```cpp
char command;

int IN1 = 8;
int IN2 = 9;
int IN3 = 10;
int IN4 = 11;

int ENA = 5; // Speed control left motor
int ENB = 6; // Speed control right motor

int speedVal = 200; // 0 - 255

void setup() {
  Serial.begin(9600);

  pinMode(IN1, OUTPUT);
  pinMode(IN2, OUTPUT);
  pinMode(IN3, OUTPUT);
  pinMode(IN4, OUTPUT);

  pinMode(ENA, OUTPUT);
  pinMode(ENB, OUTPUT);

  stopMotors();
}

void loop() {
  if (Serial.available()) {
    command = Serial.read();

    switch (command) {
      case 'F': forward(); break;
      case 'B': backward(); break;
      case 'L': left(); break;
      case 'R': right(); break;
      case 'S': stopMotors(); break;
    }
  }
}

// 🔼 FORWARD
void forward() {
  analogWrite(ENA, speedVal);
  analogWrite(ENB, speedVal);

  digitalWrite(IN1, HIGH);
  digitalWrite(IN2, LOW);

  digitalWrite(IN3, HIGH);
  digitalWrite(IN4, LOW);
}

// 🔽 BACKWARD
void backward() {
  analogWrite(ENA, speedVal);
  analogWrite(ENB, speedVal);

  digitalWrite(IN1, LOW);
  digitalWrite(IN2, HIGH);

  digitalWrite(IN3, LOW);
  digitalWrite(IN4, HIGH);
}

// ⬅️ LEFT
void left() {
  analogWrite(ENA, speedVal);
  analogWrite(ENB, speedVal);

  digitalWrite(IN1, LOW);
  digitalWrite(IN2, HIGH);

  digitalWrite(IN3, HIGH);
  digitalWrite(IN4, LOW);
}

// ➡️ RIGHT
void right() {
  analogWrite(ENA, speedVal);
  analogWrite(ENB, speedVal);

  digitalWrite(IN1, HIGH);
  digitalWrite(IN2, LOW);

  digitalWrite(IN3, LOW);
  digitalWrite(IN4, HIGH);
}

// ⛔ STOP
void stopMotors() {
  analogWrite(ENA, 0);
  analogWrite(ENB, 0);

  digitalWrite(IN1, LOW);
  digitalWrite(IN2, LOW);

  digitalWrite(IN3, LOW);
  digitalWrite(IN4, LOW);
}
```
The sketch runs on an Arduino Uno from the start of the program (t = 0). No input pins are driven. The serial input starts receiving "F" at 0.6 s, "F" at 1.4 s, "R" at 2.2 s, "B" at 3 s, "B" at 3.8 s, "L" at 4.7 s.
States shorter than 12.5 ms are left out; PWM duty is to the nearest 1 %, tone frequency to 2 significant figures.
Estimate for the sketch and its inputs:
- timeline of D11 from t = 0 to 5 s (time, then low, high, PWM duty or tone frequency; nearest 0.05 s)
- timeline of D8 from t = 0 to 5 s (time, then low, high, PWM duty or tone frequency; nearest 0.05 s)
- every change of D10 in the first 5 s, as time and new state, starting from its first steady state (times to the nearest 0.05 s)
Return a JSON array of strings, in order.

["0 s low; 2.2 s high; 4.7 s low", "0 s low; 0.6 s high; 3 s low", "0 s low; 0.6 s high; 2.2 s low; 4.7 s high"]
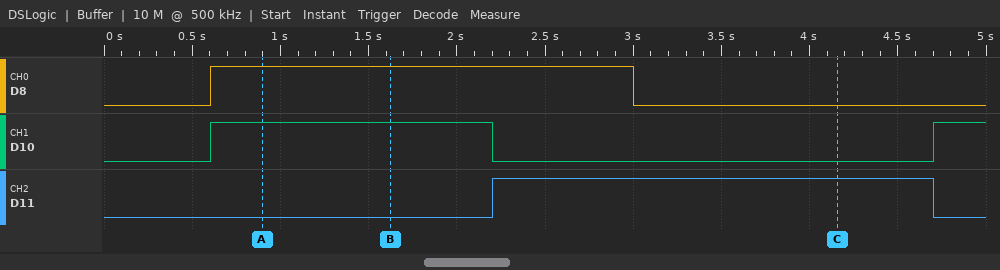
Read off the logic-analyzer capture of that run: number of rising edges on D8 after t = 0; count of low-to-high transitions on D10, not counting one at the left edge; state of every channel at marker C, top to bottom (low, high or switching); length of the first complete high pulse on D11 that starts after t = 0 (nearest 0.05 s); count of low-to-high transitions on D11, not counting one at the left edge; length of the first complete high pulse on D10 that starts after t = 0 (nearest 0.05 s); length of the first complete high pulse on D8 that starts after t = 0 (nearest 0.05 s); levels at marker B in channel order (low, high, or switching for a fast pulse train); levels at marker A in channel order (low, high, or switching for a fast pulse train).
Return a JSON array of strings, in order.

["1", "2", "D8 low, D10 low, D11 high", "2.50 s", "1", "1.60 s", "2.40 s", "D8 high, D10 high, D11 low", "D8 high, D10 high, D11 low"]
